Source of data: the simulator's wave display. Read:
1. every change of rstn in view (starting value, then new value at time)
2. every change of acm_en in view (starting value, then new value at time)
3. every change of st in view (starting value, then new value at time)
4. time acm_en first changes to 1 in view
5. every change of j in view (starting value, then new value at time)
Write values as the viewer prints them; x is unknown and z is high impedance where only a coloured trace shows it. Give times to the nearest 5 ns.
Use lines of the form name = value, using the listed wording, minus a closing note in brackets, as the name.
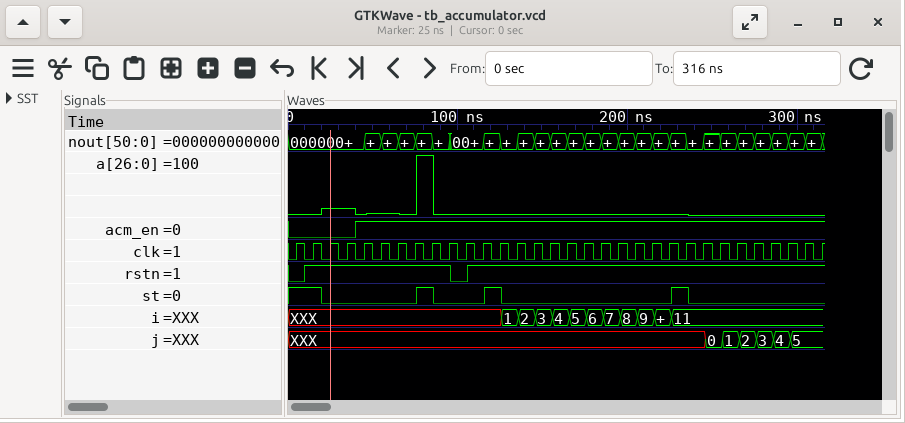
every change of rstn in view = 0, 1 at 10 ns, 0 at 95 ns, 1 at 105 ns
every change of acm_en in view = 0, 1 at 40 ns
every change of st in view = 1, 0 at 20 ns, 1 at 75 ns, 0 at 85 ns, 1 at 115 ns, 0 at 125 ns, 1 at 225 ns, 0 at 235 ns
time acm_en first changes to 1 in view = 40 ns
every change of j in view = XXX, 0 at 245 ns, 1 at 255 ns, 2 at 265 ns, 3 at 275 ns, 4 at 285 ns, 5 at 295 ns
